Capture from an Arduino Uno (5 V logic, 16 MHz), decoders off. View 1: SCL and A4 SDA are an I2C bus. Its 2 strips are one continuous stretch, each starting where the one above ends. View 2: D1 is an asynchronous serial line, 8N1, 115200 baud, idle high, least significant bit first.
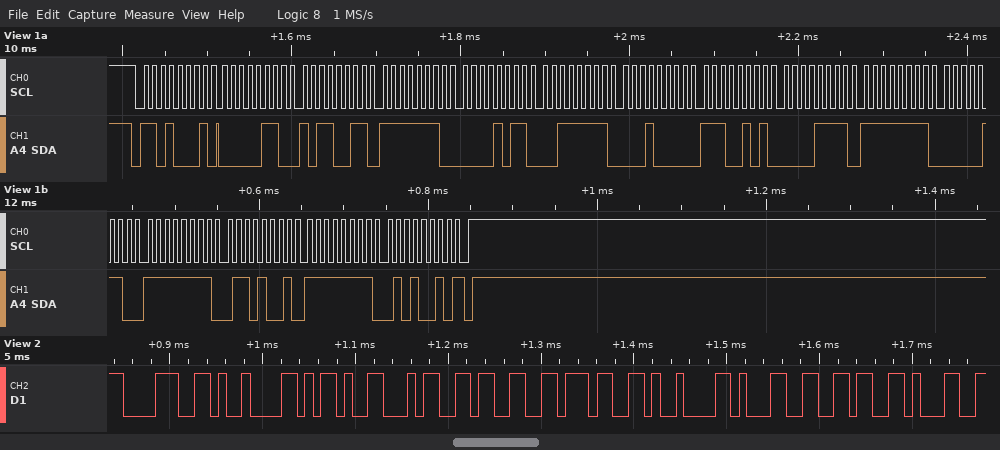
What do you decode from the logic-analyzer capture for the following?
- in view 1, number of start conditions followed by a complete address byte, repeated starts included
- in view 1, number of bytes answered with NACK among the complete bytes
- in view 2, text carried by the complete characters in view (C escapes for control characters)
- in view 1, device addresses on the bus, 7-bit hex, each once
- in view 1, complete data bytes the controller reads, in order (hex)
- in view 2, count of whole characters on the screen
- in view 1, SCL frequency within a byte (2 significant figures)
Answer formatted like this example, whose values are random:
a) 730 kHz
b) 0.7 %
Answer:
a) 1
b) 1
c) "8\t-437\t161"
d) 0x68
e) 06 B3 FE 0B 3F 10 E5 0F FF 06 FF 69 FF 52
f) 10
g) 100 kHz
